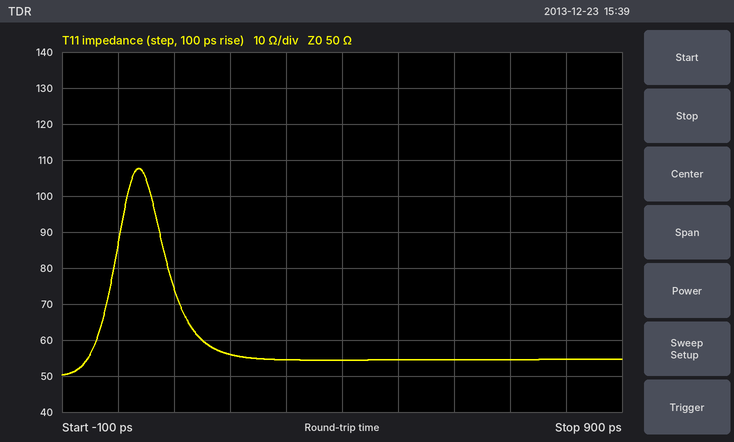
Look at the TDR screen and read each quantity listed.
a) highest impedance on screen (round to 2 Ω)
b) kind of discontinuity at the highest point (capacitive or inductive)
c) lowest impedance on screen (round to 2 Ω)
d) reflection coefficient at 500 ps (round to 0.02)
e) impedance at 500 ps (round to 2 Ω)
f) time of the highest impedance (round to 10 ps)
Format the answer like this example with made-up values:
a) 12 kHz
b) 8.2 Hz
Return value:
a) 108 Ω
b) inductive
c) 50 Ω
d) +0.04
e) 54 Ω
f) 40 ps
